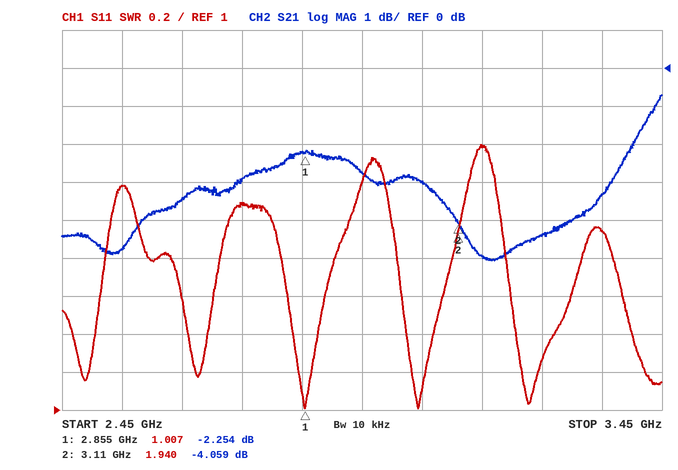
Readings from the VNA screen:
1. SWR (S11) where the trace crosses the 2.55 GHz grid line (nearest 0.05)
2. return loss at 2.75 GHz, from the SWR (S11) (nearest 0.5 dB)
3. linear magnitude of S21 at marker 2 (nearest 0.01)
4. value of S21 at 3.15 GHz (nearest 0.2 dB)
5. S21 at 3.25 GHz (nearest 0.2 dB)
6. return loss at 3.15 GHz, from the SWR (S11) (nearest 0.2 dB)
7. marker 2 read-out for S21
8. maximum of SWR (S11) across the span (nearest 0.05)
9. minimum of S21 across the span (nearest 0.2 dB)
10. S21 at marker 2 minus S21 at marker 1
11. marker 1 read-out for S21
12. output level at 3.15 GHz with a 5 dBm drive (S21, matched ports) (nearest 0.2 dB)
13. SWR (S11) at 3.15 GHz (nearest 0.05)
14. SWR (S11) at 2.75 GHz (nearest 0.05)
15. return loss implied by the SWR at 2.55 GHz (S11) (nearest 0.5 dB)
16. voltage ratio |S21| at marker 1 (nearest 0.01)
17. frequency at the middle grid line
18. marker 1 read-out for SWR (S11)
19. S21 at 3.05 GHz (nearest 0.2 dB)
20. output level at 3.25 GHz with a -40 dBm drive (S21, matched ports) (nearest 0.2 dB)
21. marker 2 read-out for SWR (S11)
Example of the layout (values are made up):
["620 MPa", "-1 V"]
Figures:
["2.20", "9.0 dB", "0.63", "-5.0 dB", "-4.4 dB", "7.8 dB", "-4.059 dB", "2.40", "-5.0 dB", "-1.805 dB", "-2.254 dB", "0.0 dBm", "2.40", "2.10", "8.5 dB", "0.77", "2.95 GHz", "1.007", "-3.0 dB", "-44.4 dBm", "1.940"]
